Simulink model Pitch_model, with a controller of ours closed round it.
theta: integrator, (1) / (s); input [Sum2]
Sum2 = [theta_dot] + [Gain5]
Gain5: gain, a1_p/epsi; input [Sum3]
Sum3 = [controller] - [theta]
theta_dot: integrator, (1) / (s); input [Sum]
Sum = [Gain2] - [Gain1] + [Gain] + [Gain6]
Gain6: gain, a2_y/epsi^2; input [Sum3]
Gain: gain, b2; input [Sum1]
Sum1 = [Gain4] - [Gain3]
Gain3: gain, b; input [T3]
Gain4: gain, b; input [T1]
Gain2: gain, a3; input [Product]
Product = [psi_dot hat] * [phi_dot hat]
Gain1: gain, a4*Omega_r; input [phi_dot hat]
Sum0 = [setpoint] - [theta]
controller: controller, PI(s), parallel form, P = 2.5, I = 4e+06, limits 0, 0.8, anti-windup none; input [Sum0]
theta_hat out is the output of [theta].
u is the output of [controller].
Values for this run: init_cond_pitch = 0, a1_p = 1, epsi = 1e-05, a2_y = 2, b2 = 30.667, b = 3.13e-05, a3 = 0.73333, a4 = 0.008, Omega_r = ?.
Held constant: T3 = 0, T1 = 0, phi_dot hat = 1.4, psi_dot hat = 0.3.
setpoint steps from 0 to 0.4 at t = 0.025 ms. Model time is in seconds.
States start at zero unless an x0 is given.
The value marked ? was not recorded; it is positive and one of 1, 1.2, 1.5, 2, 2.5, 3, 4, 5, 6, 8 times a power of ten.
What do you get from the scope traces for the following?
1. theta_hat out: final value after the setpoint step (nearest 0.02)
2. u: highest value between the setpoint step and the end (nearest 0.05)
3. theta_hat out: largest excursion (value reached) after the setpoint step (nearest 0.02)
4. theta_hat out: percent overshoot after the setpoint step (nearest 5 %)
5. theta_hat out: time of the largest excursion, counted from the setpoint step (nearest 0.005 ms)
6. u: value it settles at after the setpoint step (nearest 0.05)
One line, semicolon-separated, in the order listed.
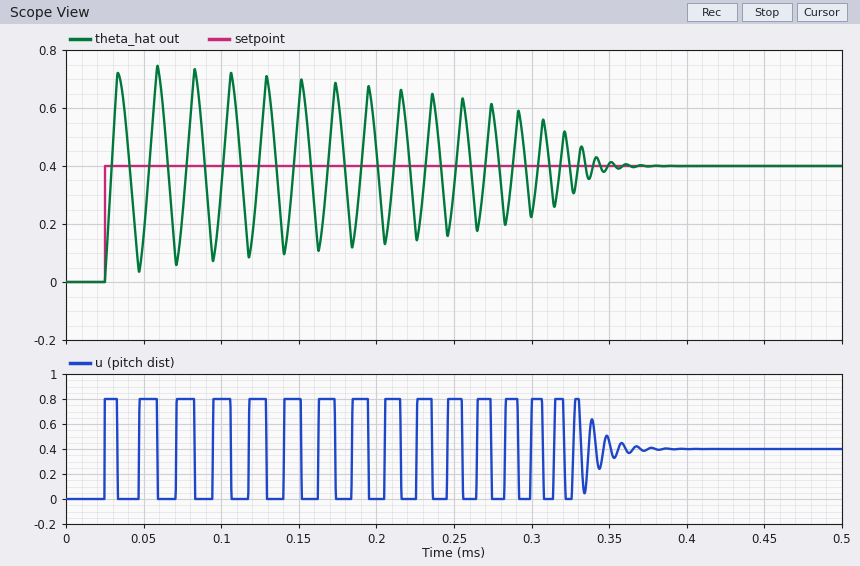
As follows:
0.40; 0.80; 0.74; 85 %; 0.035 ms; 0.40
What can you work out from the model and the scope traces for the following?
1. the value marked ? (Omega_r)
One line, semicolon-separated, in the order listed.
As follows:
0.8
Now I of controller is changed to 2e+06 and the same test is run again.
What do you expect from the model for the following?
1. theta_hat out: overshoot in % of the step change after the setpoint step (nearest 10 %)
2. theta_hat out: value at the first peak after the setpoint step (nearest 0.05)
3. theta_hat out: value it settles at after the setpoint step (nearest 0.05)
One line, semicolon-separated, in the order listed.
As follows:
70 %; 0.65; 0.40
